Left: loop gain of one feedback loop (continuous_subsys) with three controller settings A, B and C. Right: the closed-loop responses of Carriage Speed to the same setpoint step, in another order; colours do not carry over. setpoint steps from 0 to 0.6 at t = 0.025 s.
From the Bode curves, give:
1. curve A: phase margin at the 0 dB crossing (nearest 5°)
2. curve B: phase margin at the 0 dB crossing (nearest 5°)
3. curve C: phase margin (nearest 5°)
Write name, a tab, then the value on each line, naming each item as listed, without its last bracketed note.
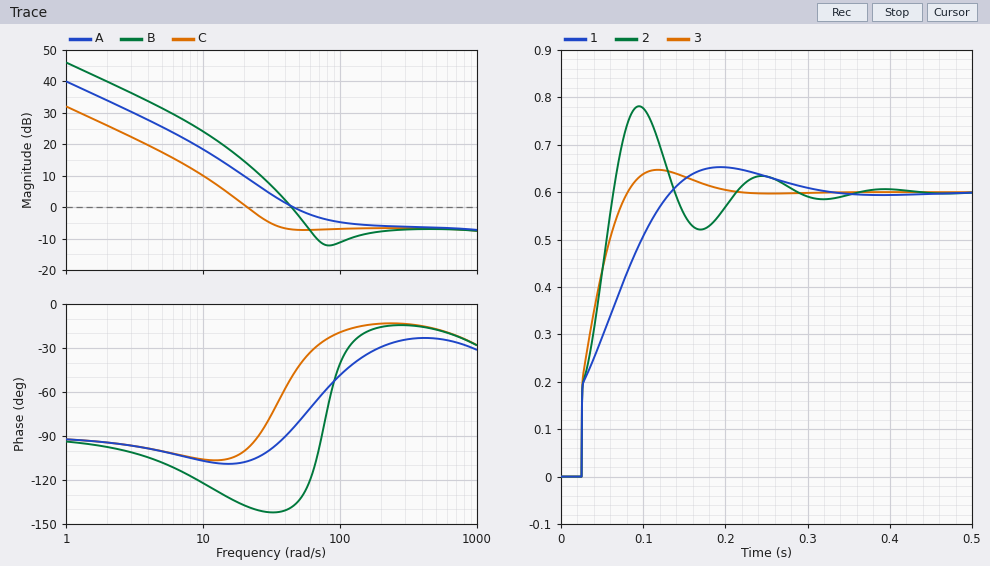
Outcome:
curve A: phase margin at the 0 dB crossing	95°
curve B: phase margin at the 0 dB crossing	40°
curve C: phase margin	80°
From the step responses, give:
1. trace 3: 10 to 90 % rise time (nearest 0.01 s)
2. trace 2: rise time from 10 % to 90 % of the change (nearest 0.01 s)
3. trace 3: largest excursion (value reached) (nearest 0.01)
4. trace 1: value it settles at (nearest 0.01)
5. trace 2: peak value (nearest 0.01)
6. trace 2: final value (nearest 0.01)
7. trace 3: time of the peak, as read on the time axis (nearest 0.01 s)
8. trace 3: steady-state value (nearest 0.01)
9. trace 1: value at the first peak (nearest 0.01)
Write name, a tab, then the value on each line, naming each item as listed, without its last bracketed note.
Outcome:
trace 3: 10 to 90 % rise time	0.04 s
trace 2: rise time from 10 % to 90 % of the change	0.03 s
trace 3: largest excursion (value reached)	0.65
trace 1: value it settles at	0.60
trace 2: peak value	0.78
trace 2: final value	0.60
trace 3: time of the peak, as read on the time axis	0.12 s
trace 3: steady-state value	0.60
trace 1: value at the first peak	0.65
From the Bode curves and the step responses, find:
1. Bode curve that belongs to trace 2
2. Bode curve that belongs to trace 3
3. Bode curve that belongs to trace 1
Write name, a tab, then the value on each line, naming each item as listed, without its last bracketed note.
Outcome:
Bode curve that belongs to trace 2	B
Bode curve that belongs to trace 3	A
Bode curve that belongs to trace 1	C
